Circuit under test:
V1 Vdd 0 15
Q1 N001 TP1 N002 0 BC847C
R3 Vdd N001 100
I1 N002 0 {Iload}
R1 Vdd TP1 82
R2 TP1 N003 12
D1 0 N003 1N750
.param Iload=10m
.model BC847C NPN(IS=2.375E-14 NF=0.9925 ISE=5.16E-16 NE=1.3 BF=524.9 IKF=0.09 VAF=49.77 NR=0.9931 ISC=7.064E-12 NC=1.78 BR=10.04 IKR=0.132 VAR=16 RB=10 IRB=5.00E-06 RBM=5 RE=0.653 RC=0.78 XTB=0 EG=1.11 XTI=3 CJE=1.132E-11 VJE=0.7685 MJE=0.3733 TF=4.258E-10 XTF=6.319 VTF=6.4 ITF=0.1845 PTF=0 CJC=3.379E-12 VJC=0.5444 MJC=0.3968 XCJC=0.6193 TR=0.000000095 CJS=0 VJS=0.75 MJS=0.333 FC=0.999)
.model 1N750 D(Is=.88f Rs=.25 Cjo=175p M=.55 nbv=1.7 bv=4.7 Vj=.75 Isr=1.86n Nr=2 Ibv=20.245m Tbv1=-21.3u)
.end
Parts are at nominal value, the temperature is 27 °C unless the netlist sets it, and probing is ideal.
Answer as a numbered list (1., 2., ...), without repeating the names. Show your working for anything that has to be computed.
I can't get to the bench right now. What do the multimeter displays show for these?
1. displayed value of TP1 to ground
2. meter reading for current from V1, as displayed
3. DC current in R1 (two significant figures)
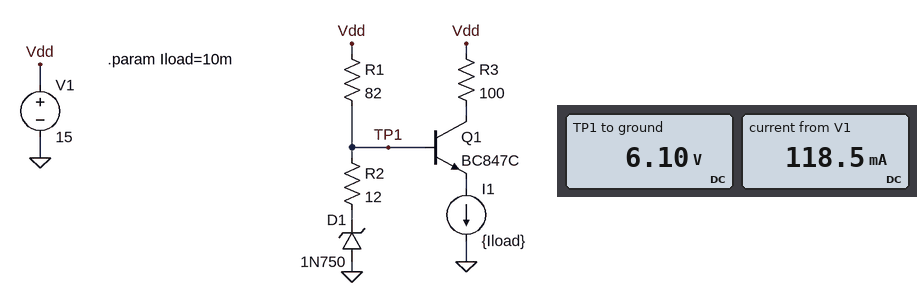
1. 6.10 V
2. 118.5 mA
3. (15 V - 6.1 V) / 82 Ω = 110 mA
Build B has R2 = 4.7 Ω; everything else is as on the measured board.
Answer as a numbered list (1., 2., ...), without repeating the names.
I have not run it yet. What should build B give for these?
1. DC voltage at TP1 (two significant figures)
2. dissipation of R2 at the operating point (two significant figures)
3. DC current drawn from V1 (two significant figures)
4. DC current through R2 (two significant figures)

1. 5.4 V
2. 65 mW
3. 130 mA
4. 120 mA
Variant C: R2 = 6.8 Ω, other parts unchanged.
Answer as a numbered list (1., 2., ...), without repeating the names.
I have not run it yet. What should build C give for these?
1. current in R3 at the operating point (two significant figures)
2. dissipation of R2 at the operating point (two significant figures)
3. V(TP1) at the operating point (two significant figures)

1. 10 mA
2. 90 mW
3. 5.6 V
